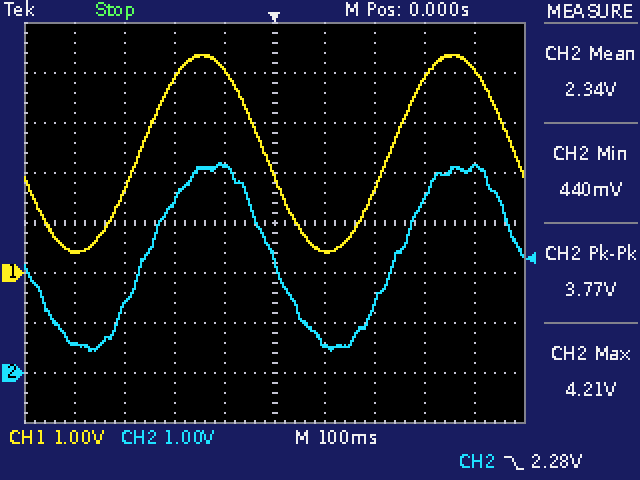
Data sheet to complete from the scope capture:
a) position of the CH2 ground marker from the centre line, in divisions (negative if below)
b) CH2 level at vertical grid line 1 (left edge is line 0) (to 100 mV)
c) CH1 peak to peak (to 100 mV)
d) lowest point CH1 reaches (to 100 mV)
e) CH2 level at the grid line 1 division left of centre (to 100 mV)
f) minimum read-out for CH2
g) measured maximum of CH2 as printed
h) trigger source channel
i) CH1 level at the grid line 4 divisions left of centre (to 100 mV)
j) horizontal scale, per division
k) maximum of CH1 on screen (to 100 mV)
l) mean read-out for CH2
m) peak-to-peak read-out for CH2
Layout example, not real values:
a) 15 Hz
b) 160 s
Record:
a) -3.0 div
b) 600 mV
c) 4.0 V
d) 400 mV
e) 4.2 V
f) 440 mV
g) 4.21 V
h) CH2
i) 400 mV
j) 100 ms
k) 4.4 V
l) 2.34 V
m) 3.77 V
